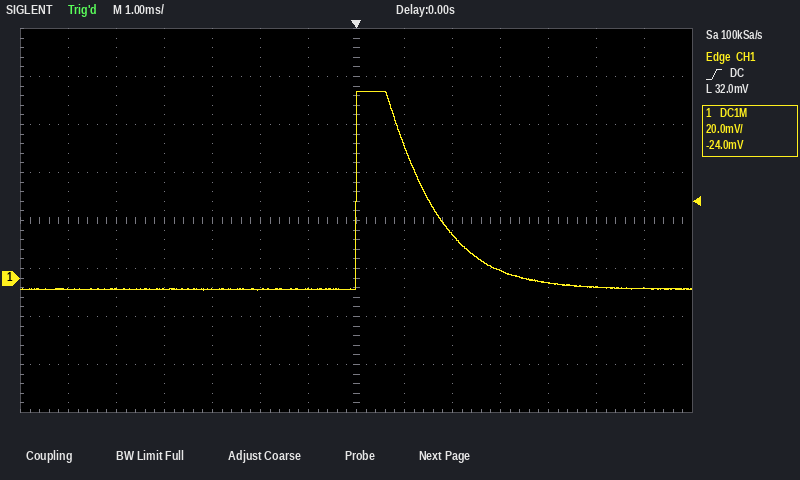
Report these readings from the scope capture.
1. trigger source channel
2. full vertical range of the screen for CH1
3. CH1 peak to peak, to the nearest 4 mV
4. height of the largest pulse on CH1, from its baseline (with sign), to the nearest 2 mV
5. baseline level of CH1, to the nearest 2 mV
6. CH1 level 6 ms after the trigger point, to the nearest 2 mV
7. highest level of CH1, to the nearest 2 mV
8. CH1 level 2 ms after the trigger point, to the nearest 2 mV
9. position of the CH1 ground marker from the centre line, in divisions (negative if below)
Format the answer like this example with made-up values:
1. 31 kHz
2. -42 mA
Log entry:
1. CH1
2. 160 mV
3. 84 mV
4. +82 mV
5. -4 mV
6. -4 mV
7. 78 mV
8. 18 mV
9. -1.2 div
